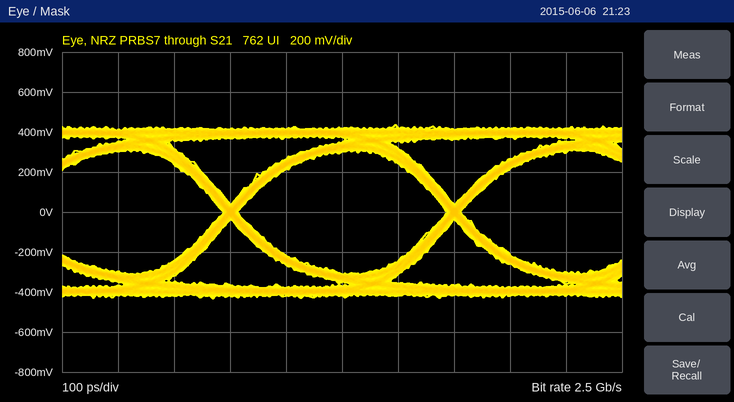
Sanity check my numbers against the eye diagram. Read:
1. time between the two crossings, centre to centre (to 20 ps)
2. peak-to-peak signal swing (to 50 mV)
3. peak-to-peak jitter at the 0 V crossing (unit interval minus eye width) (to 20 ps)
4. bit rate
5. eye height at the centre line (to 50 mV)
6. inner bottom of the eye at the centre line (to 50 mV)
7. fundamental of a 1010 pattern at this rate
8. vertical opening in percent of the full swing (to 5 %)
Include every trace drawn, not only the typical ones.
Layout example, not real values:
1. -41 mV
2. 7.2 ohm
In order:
1. 400 ps
2. 850 mV
3. 20 ps
4. 2.5 Gb/s
5. 600 mV
6. -300 mV
7. 1.25 GHz
8. 70 %
